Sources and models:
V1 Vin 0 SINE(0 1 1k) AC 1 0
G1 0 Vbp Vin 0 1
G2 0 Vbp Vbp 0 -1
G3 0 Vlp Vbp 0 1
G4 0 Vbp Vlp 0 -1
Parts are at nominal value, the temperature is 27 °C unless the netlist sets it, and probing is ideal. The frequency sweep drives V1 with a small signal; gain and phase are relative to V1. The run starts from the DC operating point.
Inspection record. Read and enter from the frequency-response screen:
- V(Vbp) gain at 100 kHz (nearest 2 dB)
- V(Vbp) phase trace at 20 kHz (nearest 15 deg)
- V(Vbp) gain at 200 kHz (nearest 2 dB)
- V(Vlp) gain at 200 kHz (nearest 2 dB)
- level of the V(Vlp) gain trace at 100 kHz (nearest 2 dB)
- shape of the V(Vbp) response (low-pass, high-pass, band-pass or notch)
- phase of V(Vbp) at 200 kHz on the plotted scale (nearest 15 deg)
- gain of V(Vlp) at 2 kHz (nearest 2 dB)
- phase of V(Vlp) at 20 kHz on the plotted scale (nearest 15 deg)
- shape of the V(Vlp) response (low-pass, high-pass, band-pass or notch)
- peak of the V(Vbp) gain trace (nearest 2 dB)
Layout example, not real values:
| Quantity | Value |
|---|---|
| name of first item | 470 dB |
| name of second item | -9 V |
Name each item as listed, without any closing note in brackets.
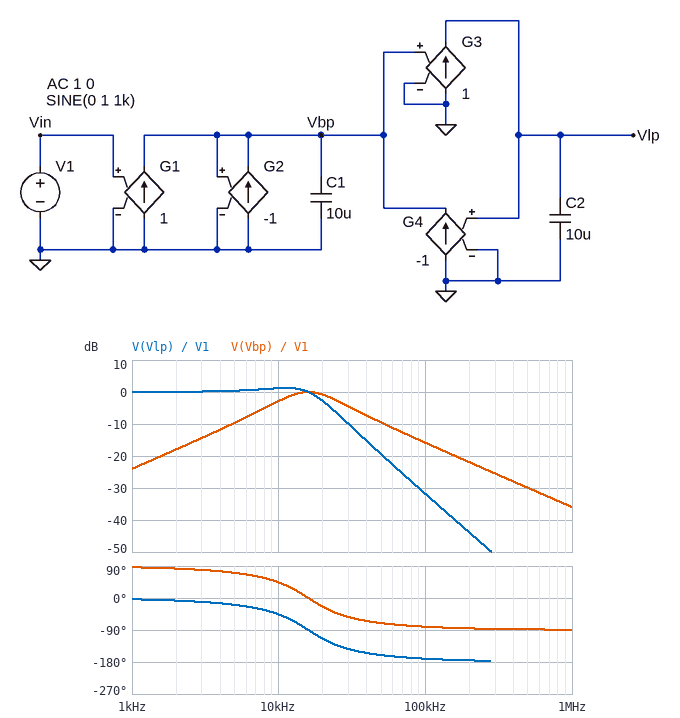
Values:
| Quantity | Value |
|---|---|
| V(Vbp) gain at 100 kHz | -16 dB |
| V(Vbp) phase trace at 20 kHz | -30 deg |
| V(Vbp) gain at 200 kHz | -22 dB |
| V(Vlp) gain at 200 kHz | -44 dB |
| level of the V(Vlp) gain trace at 100 kHz | -32 dB |
| shape of the V(Vbp) response | band-pass |
| phase of V(Vbp) at 200 kHz on the plotted scale | -90 deg |
| gain of V(Vlp) at 2 kHz | 0 dB |
| phase of V(Vlp) at 20 kHz on the plotted scale | -120 deg |
| shape of the V(Vlp) response | low-pass |
| peak of the V(Vbp) gain trace | 0 dB |
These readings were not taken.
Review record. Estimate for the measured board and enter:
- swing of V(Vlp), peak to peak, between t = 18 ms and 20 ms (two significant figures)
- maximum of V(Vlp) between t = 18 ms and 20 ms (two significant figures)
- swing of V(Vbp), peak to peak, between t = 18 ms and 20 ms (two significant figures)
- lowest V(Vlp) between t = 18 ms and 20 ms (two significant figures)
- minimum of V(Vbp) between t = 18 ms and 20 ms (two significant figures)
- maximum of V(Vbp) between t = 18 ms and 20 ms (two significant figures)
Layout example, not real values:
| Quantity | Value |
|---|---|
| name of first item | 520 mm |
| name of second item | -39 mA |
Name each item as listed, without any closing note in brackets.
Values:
| Quantity | Value |
|---|---|
| swing of V(Vlp), peak to peak, between t = 18 ms and 20 ms | 2.0 V |
| maximum of V(Vlp) between t = 18 ms and 20 ms | 1.0 V |
| swing of V(Vbp), peak to peak, between t = 18 ms and 20 ms | 130 mV |
| lowest V(Vlp) between t = 18 ms and 20 ms | -1.0 V |
| minimum of V(Vbp) between t = 18 ms and 20 ms | -63 mV |
| maximum of V(Vbp) between t = 18 ms and 20 ms | 63 mV |
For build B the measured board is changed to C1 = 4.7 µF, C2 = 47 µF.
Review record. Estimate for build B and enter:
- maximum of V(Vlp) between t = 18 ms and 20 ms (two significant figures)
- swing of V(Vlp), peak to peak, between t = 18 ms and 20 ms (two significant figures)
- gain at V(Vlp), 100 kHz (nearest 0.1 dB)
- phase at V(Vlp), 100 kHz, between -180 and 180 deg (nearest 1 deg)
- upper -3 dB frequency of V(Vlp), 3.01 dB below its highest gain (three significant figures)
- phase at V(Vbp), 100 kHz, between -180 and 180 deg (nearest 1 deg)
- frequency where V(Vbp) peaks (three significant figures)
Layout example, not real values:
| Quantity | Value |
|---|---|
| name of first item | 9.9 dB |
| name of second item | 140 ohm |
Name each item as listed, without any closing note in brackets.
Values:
| Quantity | Value |
|---|---|
| maximum of V(Vlp) between t = 18 ms and 20 ms | 970 mV |
| swing of V(Vlp), peak to peak, between t = 18 ms and 20 ms | 1.9 V |
| gain at V(Vlp), 100 kHz | -39.2 dB |
| phase at V(Vlp), 100 kHz, between -180 and 180 deg | -161 deg |
| upper -3 dB frequency of V(Vlp), 3.01 dB below its highest gain | 3.76 kHz |
| phase at V(Vbp), 100 kHz, between -180 and 180 deg | -71 deg |
| frequency where V(Vbp) peaks | 10.7 kHz |
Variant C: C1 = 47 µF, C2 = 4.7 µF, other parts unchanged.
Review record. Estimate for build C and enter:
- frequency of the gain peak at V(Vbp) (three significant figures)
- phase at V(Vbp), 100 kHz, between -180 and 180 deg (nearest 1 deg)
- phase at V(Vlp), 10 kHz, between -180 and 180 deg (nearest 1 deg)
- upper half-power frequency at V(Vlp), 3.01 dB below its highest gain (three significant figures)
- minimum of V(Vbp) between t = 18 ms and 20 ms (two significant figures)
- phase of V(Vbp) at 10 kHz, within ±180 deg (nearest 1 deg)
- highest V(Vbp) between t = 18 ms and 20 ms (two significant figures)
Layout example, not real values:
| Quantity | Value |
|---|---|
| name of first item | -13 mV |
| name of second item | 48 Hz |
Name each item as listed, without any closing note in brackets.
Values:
| Quantity | Value |
|---|---|
| frequency of the gain peak at V(Vbp) | 10.7 kHz |
| phase at V(Vbp), 100 kHz, between -180 and 180 deg | -88 deg |
| phase at V(Vlp), 10 kHz, between -180 and 180 deg | -67 deg |
| upper half-power frequency at V(Vlp), 3.01 dB below its highest gain | 12.0 kHz |
| minimum of V(Vbp) between t = 18 ms and 20 ms | -30 mV |
| phase of V(Vbp) at 10 kHz, within ±180 deg | 23 deg |
| highest V(Vbp) between t = 18 ms and 20 ms | 30 mV |
